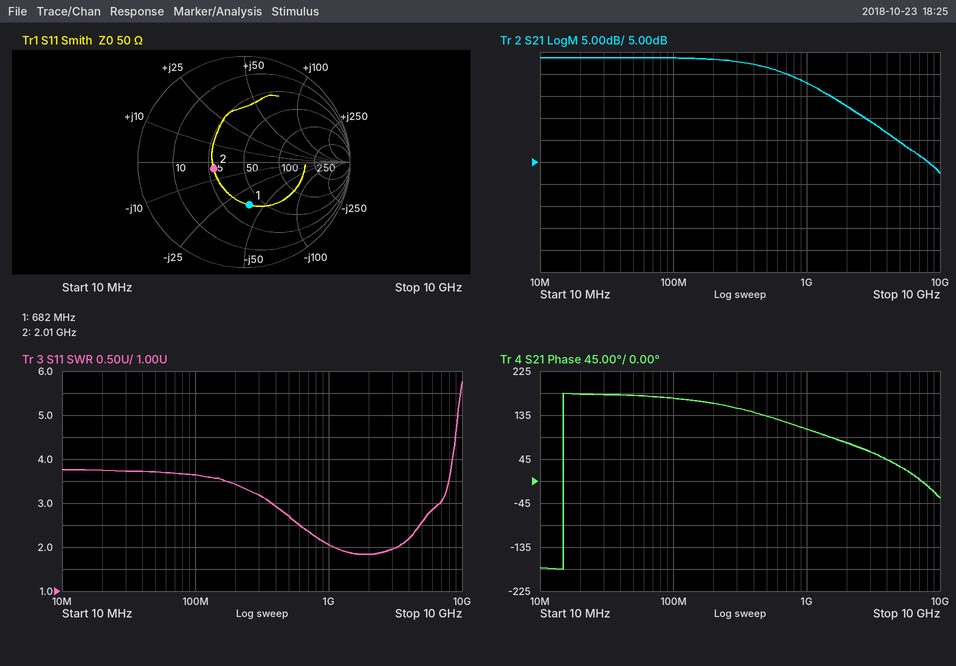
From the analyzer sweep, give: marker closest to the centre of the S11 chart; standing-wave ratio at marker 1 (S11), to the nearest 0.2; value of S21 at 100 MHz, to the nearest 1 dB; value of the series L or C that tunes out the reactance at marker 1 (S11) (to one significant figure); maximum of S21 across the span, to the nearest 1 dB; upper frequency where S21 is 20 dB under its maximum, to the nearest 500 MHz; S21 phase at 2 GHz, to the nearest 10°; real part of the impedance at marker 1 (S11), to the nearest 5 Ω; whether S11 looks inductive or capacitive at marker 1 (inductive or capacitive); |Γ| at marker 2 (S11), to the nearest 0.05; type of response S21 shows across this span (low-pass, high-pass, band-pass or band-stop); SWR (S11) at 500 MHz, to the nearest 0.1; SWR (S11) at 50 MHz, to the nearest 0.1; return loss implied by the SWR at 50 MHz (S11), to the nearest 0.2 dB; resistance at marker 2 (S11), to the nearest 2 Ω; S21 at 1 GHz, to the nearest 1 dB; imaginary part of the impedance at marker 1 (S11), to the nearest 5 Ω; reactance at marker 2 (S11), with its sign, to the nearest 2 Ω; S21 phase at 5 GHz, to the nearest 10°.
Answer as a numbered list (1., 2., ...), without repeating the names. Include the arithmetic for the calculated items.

1. marker 2
2. 2.4
3. 29 dB
4. L = 40 Ω/(2π × 682 MHz) ≈ 9 nH
5. 29 dB
6. 5.5 GHz
7. 80°
8. 40 Ω
9. capacitive
10. 0.30
11. low-pass
12. 2.7
13. 3.7
14. −20 log10((3.7 − 1)/(3.7 + 1)) ≈ 4.8 dB
15. 28 Ω
16. 23 dB
17. -40 Ω
18. -4 Ω
19. 30°
